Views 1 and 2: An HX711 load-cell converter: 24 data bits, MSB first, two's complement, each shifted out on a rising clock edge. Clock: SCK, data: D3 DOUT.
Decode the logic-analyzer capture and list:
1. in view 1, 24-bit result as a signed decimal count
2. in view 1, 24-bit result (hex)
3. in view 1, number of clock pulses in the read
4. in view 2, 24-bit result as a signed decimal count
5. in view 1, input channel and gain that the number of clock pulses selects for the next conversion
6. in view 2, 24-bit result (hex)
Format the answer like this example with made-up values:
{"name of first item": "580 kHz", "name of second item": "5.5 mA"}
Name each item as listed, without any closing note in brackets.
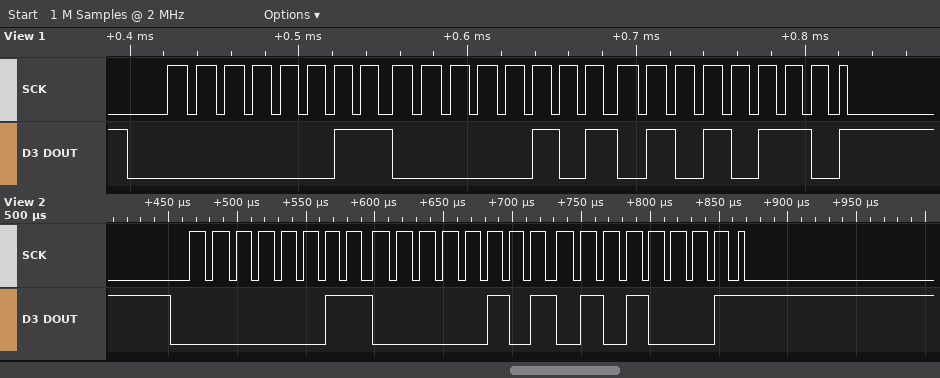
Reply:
{"in view 1, 24-bit result as a signed decimal count": "197974", "in view 1, 24-bit result": "0x030556", "in view 1, number of clock pulses in the read": "25", "in view 2, 24-bit result as a signed decimal count": "197969", "in view 1, input channel and gain that the number of clock pulses selects for the next conversion": "channel A, gain 128", "in view 2, 24-bit result": "0x030551"}
